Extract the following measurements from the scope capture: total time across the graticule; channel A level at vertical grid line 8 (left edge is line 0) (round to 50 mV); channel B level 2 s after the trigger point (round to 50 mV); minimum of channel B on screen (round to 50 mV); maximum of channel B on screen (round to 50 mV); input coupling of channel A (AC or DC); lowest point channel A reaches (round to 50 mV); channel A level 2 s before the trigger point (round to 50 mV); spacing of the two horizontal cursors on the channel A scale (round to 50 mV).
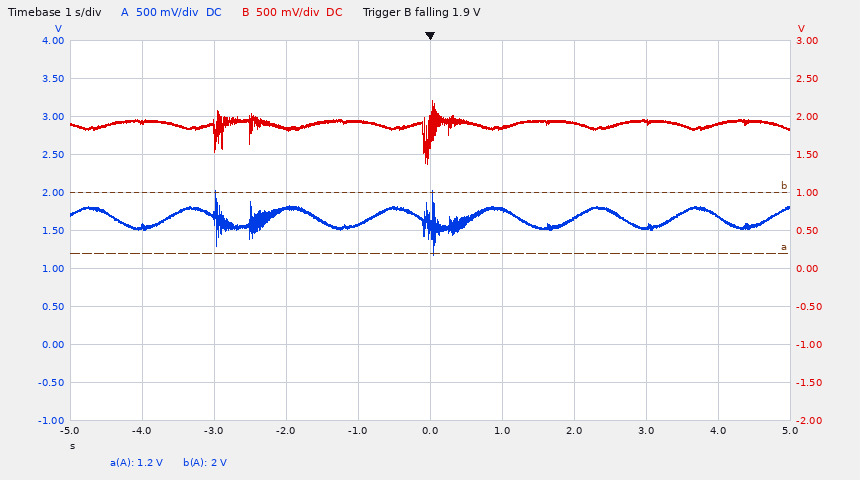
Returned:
10 s
1.55 V
1.90 V
1.40 V
2.20 V
DC
1.20 V
1.80 V
800 mV
